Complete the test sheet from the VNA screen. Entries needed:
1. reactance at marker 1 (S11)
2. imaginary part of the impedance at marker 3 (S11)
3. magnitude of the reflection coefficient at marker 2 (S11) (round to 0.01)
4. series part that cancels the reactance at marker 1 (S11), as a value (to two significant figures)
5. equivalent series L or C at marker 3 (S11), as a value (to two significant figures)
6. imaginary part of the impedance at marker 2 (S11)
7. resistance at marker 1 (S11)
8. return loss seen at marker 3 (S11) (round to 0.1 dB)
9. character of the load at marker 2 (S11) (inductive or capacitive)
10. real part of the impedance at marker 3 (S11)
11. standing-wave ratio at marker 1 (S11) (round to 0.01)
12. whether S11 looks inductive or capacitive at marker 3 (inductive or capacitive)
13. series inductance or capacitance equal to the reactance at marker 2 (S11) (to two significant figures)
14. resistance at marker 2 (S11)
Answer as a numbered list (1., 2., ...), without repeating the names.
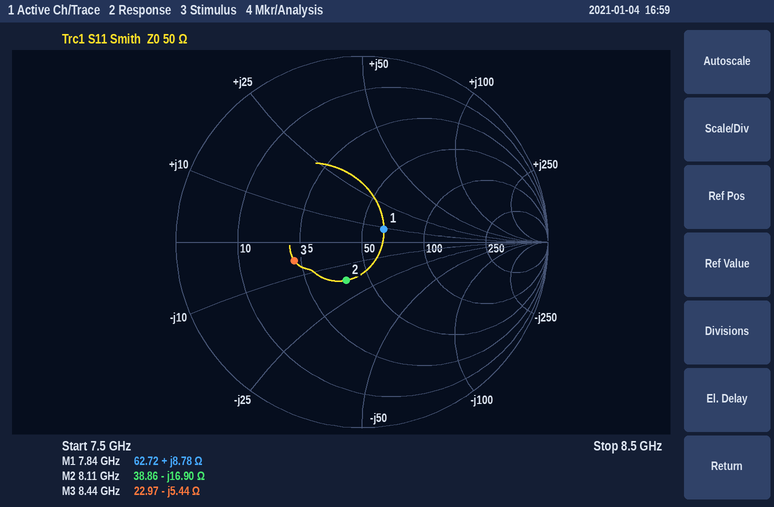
1. +8.78 Ω
2. -5.44 Ω
3. 0.22
4. 2.3 pF
5. 3.5 pF
6. -16.90 Ω
7. 62.72 Ω
8. 8.5 dB
9. capacitive
10. 22.97 Ω
11. 1.32
12. capacitive
13. 1.2 pF
14. 38.86 Ω
